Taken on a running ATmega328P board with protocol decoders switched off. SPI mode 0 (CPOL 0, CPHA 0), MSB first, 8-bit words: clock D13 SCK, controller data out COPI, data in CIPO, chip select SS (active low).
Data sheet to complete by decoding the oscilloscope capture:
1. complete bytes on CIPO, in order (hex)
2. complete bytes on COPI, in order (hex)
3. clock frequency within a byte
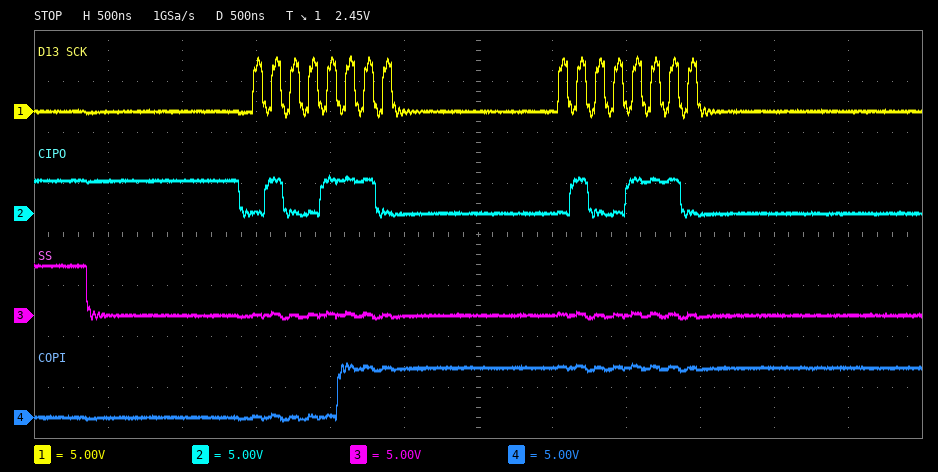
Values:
0x4E 0x4E
0x07 0xFF
8 MHz
